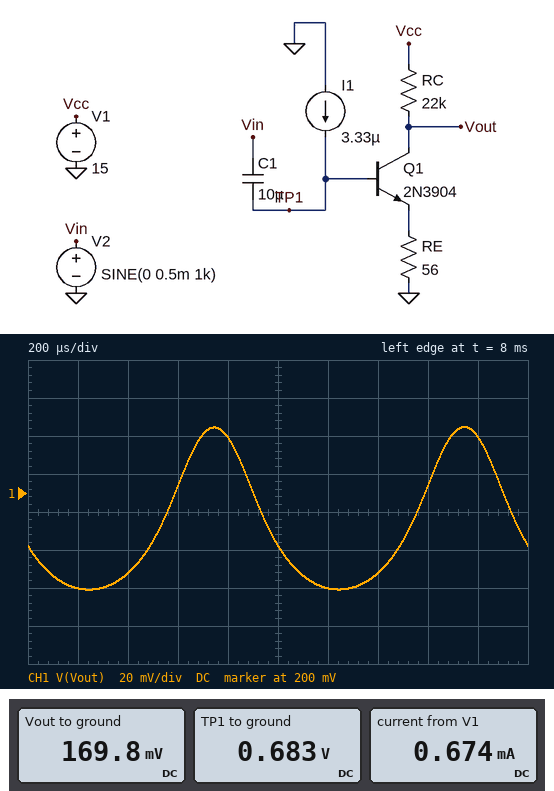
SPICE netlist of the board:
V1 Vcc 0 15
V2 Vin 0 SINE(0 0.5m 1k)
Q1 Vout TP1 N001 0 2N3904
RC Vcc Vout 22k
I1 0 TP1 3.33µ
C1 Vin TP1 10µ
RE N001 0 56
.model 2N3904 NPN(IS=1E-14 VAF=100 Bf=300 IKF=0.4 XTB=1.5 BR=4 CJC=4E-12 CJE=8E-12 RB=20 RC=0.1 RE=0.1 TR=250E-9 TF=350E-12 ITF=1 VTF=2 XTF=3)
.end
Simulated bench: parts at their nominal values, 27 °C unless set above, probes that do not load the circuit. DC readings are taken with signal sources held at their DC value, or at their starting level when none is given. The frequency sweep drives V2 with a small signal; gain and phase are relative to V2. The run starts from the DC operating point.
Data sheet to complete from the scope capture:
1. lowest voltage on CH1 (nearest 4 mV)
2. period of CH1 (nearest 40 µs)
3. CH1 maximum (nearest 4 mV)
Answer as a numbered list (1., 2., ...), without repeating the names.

1. 148 mV
2. 1.00 ms
3. 236 mV
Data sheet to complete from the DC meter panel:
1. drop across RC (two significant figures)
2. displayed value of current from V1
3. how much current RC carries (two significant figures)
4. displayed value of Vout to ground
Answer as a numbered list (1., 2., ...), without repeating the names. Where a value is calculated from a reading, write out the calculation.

1. 15 V - 169.8 mV = 15 V
2. 0.674 mA
3. (15 V - 169.8 mV) / 22 kΩ = 670 µA
4. 169.8 mV
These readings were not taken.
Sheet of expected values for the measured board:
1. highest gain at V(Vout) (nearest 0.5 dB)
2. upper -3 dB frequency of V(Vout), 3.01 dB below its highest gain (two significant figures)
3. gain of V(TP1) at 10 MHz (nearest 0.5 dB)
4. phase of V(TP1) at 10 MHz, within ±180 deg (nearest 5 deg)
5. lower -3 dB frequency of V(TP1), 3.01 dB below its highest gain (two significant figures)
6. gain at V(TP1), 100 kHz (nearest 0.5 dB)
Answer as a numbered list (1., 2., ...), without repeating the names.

1. 36.0 dB
2. 460 kHz
3. 0 dB
4. 0 deg
5. 43 Hz
6. 0 dB
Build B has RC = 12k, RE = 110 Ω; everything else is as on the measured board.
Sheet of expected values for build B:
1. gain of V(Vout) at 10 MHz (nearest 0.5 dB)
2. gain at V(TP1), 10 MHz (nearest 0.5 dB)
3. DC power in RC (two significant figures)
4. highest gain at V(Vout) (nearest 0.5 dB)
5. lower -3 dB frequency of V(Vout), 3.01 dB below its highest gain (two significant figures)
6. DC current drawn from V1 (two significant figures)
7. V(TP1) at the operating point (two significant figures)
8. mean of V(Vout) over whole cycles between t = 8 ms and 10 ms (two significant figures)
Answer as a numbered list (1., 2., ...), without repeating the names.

1. 31.0 dB
2. 0 dB
3. 12 mW
4. 38.5 dB
5. 420 mHz
6. 1.0 mA
7. 770 mV
8. 2.8 V
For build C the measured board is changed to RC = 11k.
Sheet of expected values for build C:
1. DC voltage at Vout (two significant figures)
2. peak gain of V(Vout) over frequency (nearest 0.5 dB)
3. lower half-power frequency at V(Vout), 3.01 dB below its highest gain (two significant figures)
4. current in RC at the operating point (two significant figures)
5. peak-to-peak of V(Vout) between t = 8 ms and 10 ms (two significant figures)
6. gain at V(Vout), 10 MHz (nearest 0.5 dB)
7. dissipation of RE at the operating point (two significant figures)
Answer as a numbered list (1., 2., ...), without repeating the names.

1. 3.7 V
2. 42.5 dB
3. 680 mHz
4. 1.0 mA
5. 130 mV
6. 35.5 dB
7. 59 µW
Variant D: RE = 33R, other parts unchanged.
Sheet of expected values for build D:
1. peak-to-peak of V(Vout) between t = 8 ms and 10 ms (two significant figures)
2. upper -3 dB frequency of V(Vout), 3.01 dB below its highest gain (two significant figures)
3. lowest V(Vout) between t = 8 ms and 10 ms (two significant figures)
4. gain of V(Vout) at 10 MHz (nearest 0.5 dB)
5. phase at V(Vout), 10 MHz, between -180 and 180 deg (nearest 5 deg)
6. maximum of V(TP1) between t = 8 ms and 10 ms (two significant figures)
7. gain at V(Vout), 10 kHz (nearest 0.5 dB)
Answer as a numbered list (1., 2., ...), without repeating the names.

1. 110 mV
2. 500 kHz
3. 130 mV
4. 11.5 dB
5. 80 deg
6. 670 mV
7. 37.5 dB
